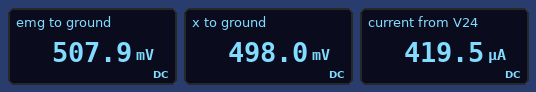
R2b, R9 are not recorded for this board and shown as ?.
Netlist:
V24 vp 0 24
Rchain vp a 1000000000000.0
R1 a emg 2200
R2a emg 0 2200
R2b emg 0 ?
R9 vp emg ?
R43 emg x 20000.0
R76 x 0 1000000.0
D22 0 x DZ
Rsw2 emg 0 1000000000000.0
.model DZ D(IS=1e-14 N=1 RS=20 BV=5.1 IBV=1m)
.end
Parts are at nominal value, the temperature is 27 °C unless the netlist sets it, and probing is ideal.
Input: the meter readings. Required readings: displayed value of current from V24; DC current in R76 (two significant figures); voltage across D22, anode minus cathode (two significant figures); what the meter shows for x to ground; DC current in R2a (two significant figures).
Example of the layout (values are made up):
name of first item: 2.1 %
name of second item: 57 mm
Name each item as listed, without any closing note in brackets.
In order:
displayed value of current from V24: 419.5 µA
DC current in R76: 500 nA
voltage across D22, anode minus cathode: -500 mV
what the meter shows for x to ground: 498.0 mV
DC current in R2a: 230 µA
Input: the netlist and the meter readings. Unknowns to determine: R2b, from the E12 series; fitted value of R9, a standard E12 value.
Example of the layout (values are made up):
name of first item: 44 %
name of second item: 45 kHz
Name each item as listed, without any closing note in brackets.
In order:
R2b, from the E12 series: 2.7 kΩ
fitted value of R9, a standard E12 value: 56 kΩ
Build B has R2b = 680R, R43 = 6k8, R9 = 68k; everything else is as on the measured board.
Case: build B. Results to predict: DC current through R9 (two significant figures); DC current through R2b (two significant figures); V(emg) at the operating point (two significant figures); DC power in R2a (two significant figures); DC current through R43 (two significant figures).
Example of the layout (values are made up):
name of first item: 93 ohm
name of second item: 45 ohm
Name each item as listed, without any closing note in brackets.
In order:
DC current through R9: 350 µA
DC current through R2b: 270 µA
V(emg) at the operating point: 180 mV
DC power in R2a: 15 µW
DC current through R43: 180 nA
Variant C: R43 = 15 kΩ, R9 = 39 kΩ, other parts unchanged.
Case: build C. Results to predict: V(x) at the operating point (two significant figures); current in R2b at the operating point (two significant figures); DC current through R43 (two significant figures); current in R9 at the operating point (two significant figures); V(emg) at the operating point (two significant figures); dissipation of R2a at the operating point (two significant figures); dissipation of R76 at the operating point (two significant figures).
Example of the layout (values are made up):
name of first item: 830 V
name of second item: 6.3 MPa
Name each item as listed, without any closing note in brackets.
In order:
V(x) at the operating point: 710 mV
current in R2b at the operating point: 270 µA
DC current through R43: 710 nA
current in R9 at the operating point: 600 µA
V(emg) at the operating point: 720 mV
dissipation of R2a at the operating point: 240 µW
dissipation of R76 at the operating point: 510 nW
